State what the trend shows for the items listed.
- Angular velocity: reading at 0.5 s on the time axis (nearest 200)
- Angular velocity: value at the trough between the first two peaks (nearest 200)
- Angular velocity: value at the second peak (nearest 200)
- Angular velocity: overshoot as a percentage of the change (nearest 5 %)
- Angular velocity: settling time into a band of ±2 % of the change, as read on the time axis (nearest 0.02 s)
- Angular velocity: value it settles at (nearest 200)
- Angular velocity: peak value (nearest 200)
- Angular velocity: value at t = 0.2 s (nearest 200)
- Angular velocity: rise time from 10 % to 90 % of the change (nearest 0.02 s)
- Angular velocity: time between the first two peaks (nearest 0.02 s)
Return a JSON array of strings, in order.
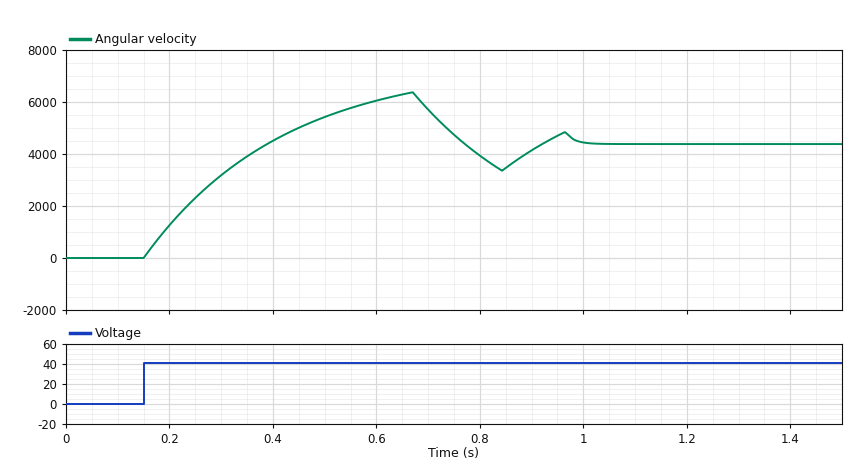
["5400", "3400", "4800", "45 %", "1.00 s", "4400", "6400", "1200", "0.18 s", "0.30 s"]
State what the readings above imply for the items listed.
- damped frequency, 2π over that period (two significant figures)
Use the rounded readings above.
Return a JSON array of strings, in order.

["21 rad/s"]
